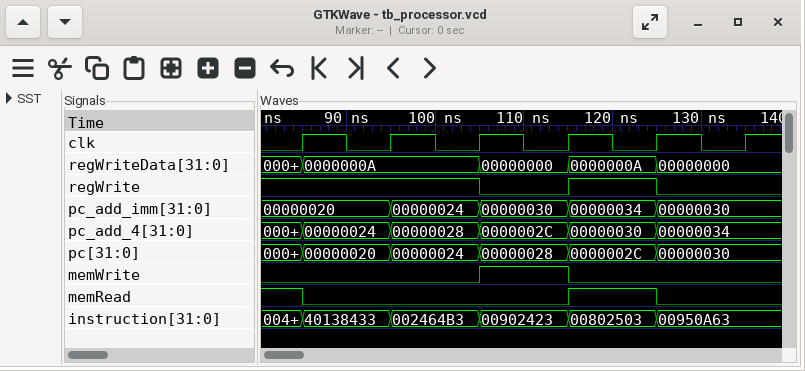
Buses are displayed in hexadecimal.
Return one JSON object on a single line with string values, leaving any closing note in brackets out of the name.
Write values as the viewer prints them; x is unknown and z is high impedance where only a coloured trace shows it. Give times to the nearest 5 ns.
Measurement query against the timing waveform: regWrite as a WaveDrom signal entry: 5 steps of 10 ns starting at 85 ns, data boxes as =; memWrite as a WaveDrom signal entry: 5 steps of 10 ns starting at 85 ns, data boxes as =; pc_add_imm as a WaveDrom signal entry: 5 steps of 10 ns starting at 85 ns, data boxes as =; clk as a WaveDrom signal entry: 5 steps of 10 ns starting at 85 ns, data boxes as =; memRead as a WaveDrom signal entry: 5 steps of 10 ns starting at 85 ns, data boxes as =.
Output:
{"regWrite as a WaveDrom signal entry: 5 steps of 10 ns starting at 85 ns, data boxes as =": "{name: 'regWrite', wave: '1.010'}", "memWrite as a WaveDrom signal entry: 5 steps of 10 ns starting at 85 ns, data boxes as =": "{name: 'memWrite', wave: '0.10.'}", "pc_add_imm as a WaveDrom signal entry: 5 steps of 10 ns starting at 85 ns, data boxes as =": "{name: 'pc_add_imm', wave: '=====', data: '00000020 00000024 00000030 00000034 00000030'}", "clk as a WaveDrom signal entry: 5 steps of 10 ns starting at 85 ns, data boxes as =": "{name: 'clk', wave: 'p....'}", "memRead as a WaveDrom signal entry: 5 steps of 10 ns starting at 85 ns, data boxes as =": "{name: 'memRead', wave: '0..10'}"}
